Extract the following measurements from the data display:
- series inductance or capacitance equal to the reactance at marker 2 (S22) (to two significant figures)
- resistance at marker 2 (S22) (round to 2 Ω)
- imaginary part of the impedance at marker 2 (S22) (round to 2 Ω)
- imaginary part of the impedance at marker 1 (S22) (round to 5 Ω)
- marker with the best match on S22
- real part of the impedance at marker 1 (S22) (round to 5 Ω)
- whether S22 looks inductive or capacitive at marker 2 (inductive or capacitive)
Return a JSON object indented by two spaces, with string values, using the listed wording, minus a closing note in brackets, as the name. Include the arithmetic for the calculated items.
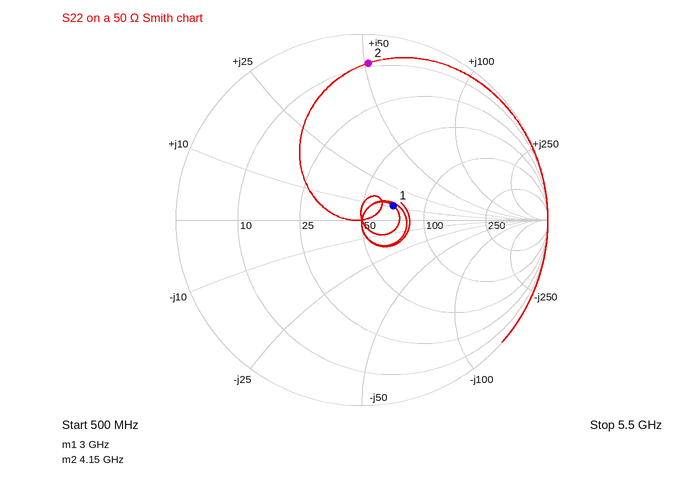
{
  "series inductance or capacitance equal to the reactance at marker 2 (S22)": "L = 52 Ω/(2π × 4.15 GHz) ≈ 2.0 nH",
  "resistance at marker 2 (S22)": "8 Ω",
  "imaginary part of the impedance at marker 2 (S22)": "+52 Ω",
  "imaginary part of the impedance at marker 1 (S22)": "+10 Ω",
  "marker with the best match on S22": "marker 1",
  "real part of the impedance at marker 1 (S22)": "70 Ω",
  "whether S22 looks inductive or capacitive at marker 2": "inductive"
}
